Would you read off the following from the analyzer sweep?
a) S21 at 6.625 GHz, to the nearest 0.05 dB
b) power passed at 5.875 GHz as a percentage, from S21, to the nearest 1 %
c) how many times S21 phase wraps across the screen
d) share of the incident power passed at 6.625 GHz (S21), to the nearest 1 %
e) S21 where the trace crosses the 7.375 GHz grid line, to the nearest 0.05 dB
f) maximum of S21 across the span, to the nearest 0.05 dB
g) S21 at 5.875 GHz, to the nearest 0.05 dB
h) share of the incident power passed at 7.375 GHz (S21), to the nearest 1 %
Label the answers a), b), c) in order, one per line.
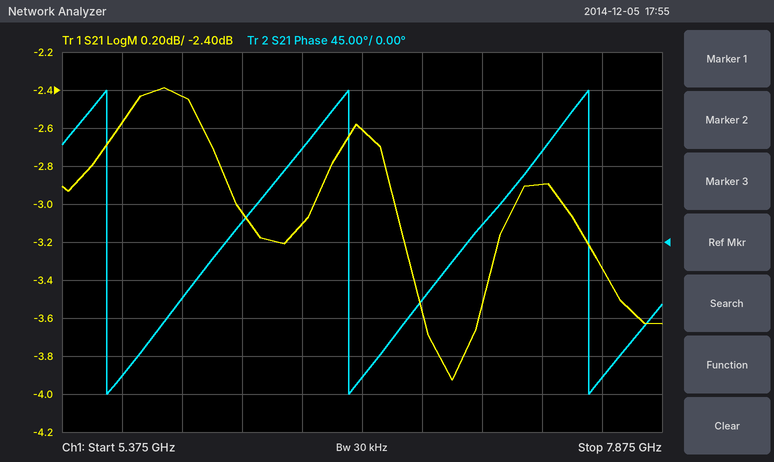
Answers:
a) -2.60 dB
b) 57 %
c) 3
d) 55 %
e) -2.90 dB
f) -2.40 dB
g) -2.45 dB
h) 51 %
